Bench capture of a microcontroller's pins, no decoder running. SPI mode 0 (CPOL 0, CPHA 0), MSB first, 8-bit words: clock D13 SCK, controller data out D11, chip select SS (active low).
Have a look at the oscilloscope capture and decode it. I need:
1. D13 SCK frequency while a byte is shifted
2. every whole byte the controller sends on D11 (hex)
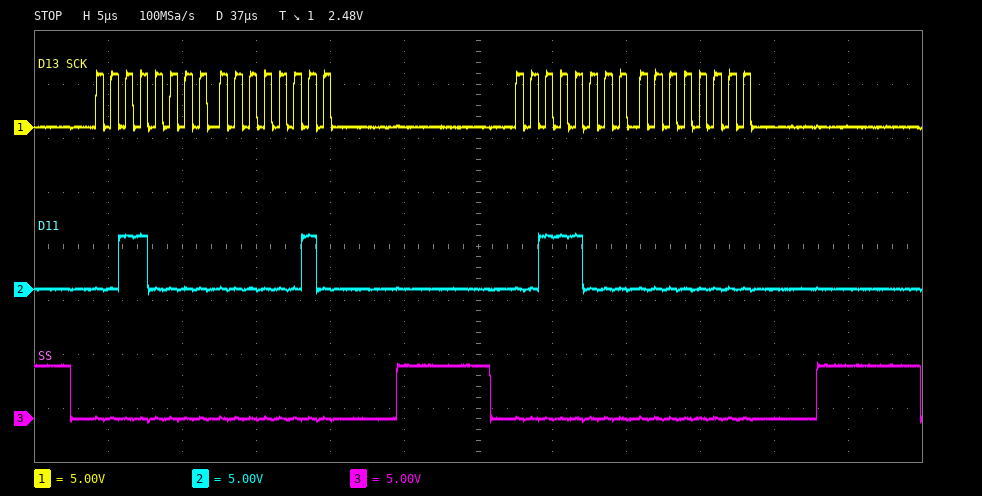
1 MHz
0x30 0x02 0x38 0x00
